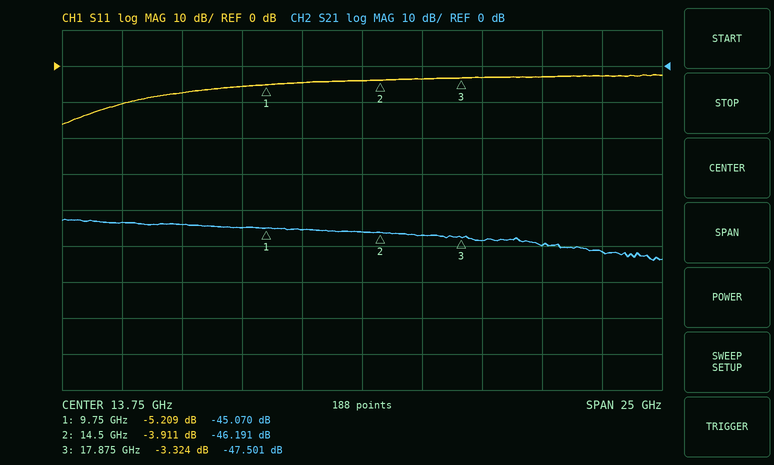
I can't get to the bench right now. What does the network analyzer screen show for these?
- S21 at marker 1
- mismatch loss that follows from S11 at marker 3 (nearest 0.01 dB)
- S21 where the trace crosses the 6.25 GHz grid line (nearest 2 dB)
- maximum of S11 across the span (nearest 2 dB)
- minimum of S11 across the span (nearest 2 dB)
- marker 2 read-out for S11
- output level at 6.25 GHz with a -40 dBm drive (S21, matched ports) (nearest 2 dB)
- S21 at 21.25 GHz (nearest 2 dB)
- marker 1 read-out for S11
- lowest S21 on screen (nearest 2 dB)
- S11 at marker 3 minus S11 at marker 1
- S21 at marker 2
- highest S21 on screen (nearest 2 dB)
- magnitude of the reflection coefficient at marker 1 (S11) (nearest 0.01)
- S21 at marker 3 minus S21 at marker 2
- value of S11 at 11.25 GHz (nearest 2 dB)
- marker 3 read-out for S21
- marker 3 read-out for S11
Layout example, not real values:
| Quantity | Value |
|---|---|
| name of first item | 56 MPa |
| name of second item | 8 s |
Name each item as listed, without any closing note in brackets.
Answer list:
| Quantity | Value |
|---|---|
| S21 at marker 1 | -45.070 dB |
| mismatch loss that follows from S11 at marker 3 | 2.72 dB |
| S21 where the trace crosses the 6.25 GHz grid line | -44 dB |
| maximum of S11 across the span | -2 dB |
| minimum of S11 across the span | -16 dB |
| marker 2 read-out for S11 | -3.911 dB |
| output level at 6.25 GHz with a -40 dBm drive (S21, matched ports) | -84 dBm |
| S21 at 21.25 GHz | -50 dB |
| marker 1 read-out for S11 | -5.209 dB |
| lowest S21 on screen | -54 dB |
| S11 at marker 3 minus S11 at marker 1 | 1.885 dB |
| S21 at marker 2 | -46.191 dB |
| highest S21 on screen | -42 dB |
| magnitude of the reflection coefficient at marker 1 (S11) | 0.55 |
| S21 at marker 3 minus S21 at marker 2 | -1.310 dB |
| value of S11 at 11.25 GHz | -4 dB |
| marker 3 read-out for S21 | -47.501 dB |
| marker 3 read-out for S11 | -3.324 dB |
